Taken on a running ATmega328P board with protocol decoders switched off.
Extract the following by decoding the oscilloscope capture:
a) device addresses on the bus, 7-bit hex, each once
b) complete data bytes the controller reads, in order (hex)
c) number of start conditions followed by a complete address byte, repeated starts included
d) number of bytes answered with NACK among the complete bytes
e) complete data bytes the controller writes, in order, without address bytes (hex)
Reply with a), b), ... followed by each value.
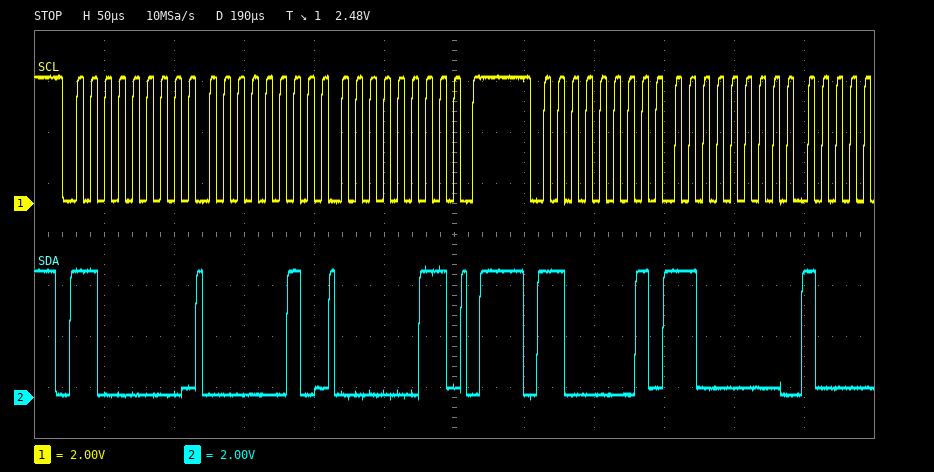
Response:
a) 0x60
b) C0
c) 2
d) 0
e) 02 03
